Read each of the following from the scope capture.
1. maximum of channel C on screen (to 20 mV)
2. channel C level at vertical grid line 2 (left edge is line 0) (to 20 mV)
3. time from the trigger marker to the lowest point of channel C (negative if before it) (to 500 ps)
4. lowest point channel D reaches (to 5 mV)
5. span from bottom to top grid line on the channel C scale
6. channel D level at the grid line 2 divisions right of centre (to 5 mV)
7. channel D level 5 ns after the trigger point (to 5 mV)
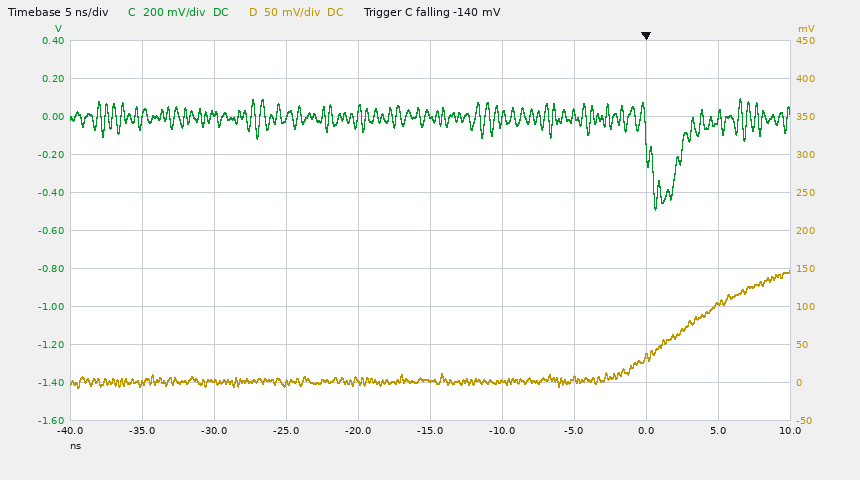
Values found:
100 mV
20 mV
+500 ps
-5 mV
2 V
5 mV
105 mV
